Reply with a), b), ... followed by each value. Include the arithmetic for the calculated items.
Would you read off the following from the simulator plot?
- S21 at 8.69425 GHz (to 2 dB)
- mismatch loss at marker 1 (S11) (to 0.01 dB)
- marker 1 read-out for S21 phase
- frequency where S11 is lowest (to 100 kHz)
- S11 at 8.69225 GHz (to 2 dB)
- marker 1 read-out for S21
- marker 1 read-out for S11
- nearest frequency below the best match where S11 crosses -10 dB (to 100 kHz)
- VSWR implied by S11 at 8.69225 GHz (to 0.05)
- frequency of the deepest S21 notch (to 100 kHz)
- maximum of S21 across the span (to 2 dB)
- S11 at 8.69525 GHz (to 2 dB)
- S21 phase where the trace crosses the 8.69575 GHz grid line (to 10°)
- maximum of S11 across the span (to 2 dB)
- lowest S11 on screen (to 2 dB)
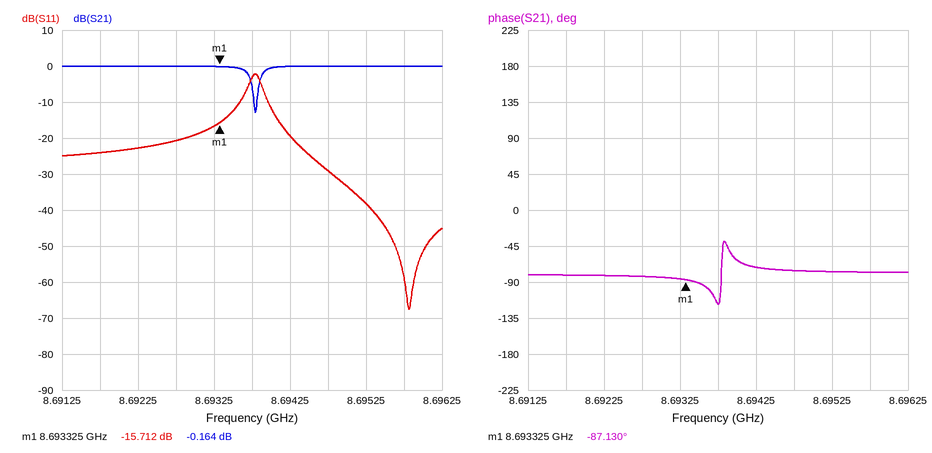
a) 0 dB
b) −10 log10(1 − 10^(-15.712/10)) ≈ 0.12 dB
c) -87.130°
d) 8.6958 GHz
e) -22 dB
f) -0.164 dB
g) -15.712 dB
h) 8.6940 GHz
i) |Γ| = 10^(-22/20) = 0.0794; VSWR = (1 + 0.0794)/(1 − 0.0794) ≈ 1.17, so 1.15 to the nearest 0.05
j) 8.6938 GHz
k) 0 dB
l) -38 dB
m) -80°
n) -2 dB
o) -68 dB
